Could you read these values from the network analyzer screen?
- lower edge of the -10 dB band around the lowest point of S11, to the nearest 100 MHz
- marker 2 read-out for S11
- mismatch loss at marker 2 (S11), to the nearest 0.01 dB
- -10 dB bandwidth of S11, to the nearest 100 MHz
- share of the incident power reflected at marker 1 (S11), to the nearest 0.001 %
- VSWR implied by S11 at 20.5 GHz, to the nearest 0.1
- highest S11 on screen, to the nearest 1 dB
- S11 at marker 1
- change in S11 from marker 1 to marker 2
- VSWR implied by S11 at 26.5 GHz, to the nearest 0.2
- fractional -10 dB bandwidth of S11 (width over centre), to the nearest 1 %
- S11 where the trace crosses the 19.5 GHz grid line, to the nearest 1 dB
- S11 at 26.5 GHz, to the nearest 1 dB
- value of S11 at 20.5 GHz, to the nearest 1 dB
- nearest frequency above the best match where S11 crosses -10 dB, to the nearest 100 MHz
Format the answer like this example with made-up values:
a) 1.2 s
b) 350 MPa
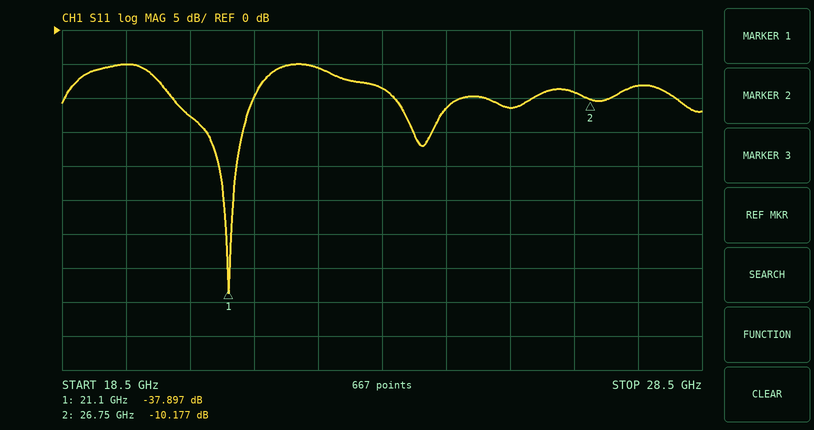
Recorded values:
a) 20.2 GHz
b) -10.177 dB
c) 0.44 dB
d) 1.3 GHz
e) 0.016 %
f) 1.6
g) -5 dB
h) -37.897 dB
i) 27.720 dB
j) 2.0
k) 6 %
l) -5 dB
m) -9 dB
n) -13 dB
o) 21.5 GHz
